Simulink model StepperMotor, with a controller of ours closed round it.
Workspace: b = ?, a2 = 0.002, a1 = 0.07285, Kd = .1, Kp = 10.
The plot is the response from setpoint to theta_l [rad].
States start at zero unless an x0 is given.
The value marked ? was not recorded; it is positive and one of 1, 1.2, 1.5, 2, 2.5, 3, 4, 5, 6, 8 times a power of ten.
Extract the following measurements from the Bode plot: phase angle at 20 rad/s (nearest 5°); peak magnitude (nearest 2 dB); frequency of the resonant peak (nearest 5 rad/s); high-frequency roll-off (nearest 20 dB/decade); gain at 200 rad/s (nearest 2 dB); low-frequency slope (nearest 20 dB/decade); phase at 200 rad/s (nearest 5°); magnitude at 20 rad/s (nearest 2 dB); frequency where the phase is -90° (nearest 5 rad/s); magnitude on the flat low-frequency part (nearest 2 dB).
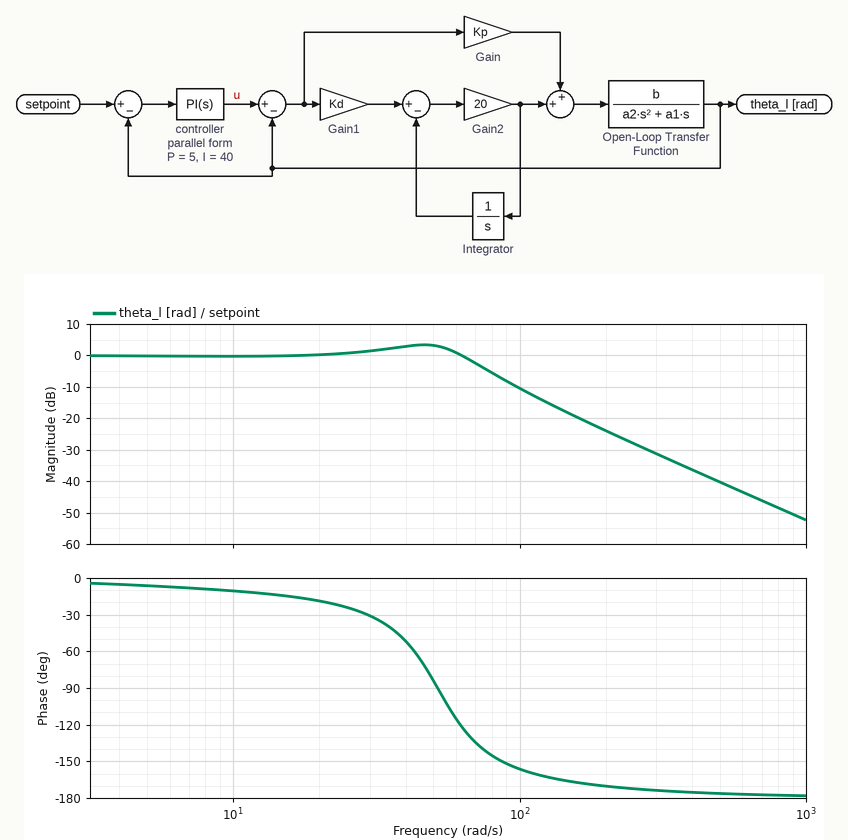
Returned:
-20°
4 dB
45 rad/s
-40 dB/decade
-24 dB
0 dB/decade
-170°
0 dB
50 rad/s
0 dB
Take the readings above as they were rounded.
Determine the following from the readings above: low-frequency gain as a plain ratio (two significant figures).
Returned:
1.0
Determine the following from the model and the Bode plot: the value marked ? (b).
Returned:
0.08
